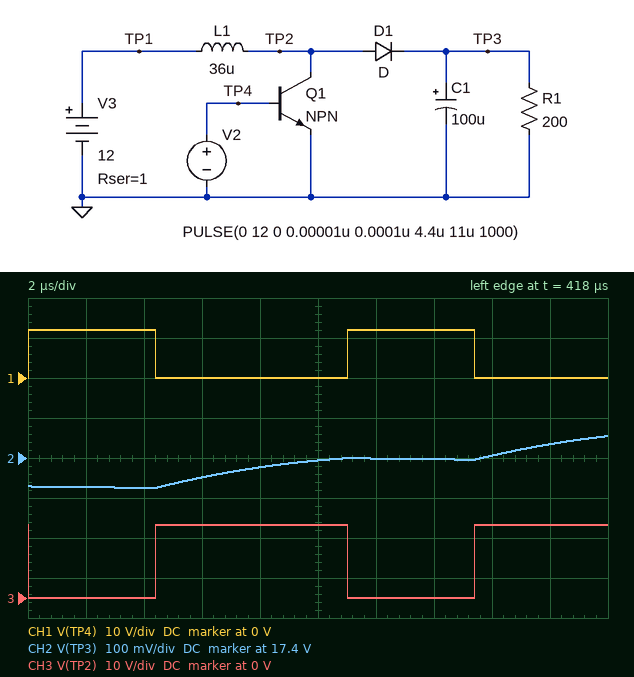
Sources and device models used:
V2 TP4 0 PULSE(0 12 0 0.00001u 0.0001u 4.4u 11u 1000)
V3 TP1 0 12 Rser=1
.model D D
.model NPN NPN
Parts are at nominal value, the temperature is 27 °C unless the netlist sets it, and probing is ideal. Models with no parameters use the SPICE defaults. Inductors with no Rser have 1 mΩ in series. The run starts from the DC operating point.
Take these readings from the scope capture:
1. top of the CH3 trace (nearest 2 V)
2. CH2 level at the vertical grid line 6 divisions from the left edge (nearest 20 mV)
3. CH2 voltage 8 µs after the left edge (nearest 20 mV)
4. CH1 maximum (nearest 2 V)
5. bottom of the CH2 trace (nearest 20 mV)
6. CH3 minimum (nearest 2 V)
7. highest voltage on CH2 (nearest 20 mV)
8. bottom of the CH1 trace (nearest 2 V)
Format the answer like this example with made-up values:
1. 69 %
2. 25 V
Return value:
1. 18 V
2. 17.40 V
3. 17.38 V
4. 12 V
5. 17.32 V
6. 0 V
7. 17.46 V
8. 0 V
